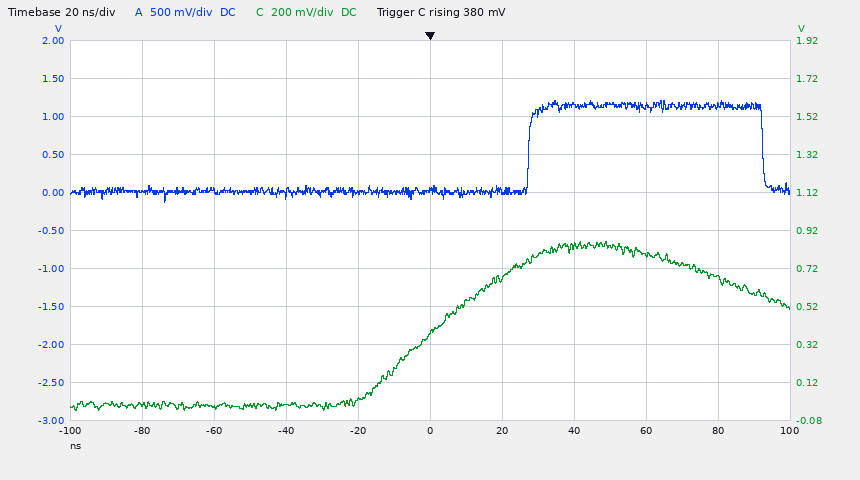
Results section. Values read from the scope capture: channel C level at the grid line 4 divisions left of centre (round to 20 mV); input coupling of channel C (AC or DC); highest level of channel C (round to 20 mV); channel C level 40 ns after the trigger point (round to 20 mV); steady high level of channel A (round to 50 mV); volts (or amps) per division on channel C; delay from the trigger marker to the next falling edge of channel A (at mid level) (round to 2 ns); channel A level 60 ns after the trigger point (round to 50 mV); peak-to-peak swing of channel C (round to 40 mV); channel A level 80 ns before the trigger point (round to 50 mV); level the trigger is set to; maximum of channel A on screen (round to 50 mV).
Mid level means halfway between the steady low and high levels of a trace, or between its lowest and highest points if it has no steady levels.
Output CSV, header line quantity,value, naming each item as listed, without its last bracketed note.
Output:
quantity,value
channel C level at the grid line 4 divisions left of centre,0 mV
input coupling of channel C,DC
highest level of channel C,860 mV
channel C level 40 ns after the trigger point,840 mV
steady high level of channel A,1.15 V
volts (or amps) per division on channel C,200 mV
delay from the trigger marker to the next falling edge of channel A (at mid level),92 ns
channel A level 60 ns after the trigger point,1.15 V
peak-to-peak swing of channel C,880 mV
channel A level 80 ns before the trigger point,0 mV
level the trigger is set to,380 mV
maximum of channel A on screen,1.20 V
